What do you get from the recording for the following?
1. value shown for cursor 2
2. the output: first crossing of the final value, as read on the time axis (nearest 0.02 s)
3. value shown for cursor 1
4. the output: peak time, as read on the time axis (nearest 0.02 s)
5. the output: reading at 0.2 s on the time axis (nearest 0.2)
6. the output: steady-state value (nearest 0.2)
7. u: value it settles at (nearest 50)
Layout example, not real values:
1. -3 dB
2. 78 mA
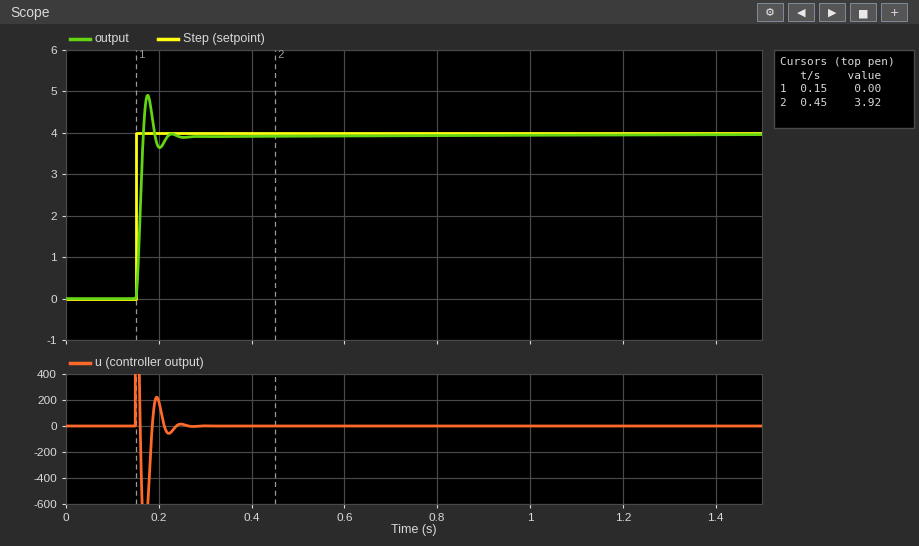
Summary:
1. 3.92
2. 0.16 s
3. 0.00
4. 0.18 s
5. 3.6
6. 4.0
7. 0
